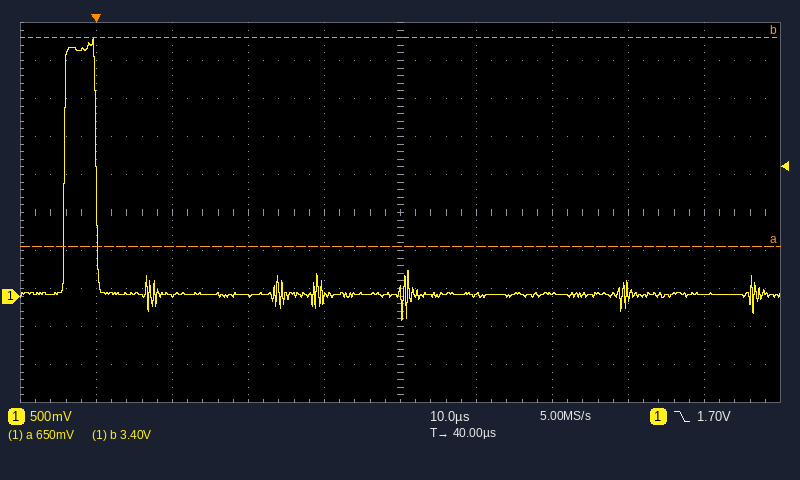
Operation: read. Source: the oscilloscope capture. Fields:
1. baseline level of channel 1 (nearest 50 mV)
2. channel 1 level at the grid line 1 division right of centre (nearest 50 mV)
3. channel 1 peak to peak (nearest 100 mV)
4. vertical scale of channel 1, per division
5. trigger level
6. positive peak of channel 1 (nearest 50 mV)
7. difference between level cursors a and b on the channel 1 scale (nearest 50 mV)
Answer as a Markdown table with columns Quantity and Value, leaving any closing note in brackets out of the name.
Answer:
| Quantity | Value |
|---|---|
| baseline level of channel 1 | 0 mV |
| channel 1 level at the grid line 1 division right of centre | 0 mV |
| channel 1 peak to peak | 3.70 V |
| vertical scale of channel 1, per division | 500 mV |
| trigger level | 1.70 V |
| positive peak of channel 1 | 3.40 V |
| difference between level cursors a and b on the channel 1 scale | 2.75 V |
